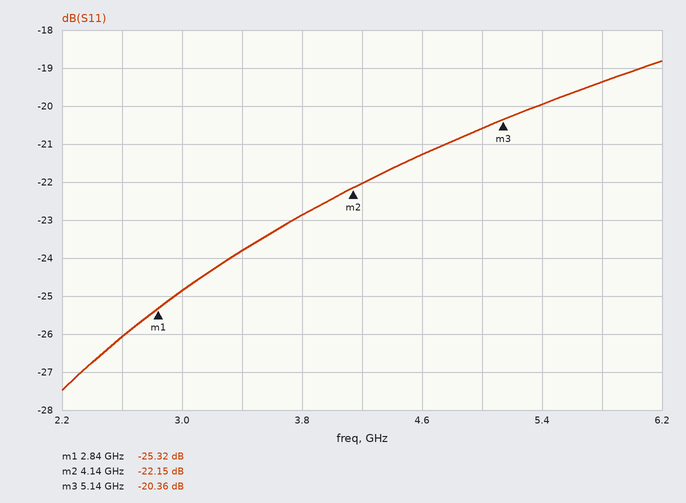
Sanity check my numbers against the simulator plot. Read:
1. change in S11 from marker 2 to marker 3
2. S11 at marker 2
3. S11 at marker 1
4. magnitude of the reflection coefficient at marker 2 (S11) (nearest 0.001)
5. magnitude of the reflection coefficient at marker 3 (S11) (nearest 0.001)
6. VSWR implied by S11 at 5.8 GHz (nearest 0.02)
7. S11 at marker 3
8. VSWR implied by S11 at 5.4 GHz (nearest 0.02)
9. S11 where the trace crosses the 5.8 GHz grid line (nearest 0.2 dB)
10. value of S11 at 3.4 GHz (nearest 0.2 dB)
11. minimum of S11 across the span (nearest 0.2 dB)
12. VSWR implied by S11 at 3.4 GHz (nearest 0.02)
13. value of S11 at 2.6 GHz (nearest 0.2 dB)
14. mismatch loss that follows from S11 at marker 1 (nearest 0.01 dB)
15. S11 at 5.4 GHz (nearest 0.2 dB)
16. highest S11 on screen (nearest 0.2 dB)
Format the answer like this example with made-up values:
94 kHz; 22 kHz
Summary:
1.79 dB; -22.15 dB; -25.32 dB; 0.078; 0.096; 1.24; -20.36 dB; 1.22; -19.4 dB; -23.8 dB; -27.4 dB; 1.14; -26.0 dB; 0.01 dB; -20.0 dB; -18.8 dB
